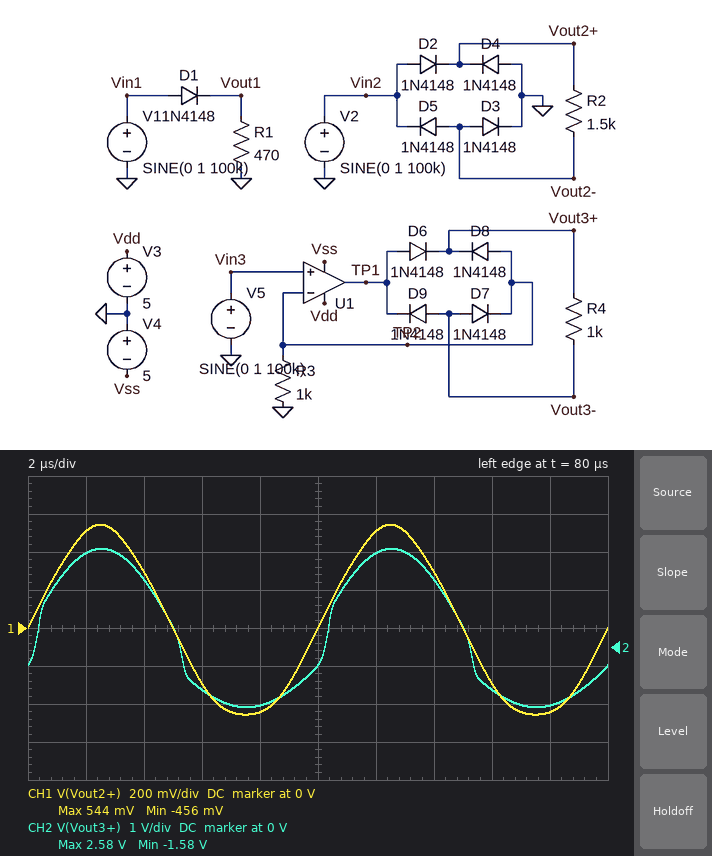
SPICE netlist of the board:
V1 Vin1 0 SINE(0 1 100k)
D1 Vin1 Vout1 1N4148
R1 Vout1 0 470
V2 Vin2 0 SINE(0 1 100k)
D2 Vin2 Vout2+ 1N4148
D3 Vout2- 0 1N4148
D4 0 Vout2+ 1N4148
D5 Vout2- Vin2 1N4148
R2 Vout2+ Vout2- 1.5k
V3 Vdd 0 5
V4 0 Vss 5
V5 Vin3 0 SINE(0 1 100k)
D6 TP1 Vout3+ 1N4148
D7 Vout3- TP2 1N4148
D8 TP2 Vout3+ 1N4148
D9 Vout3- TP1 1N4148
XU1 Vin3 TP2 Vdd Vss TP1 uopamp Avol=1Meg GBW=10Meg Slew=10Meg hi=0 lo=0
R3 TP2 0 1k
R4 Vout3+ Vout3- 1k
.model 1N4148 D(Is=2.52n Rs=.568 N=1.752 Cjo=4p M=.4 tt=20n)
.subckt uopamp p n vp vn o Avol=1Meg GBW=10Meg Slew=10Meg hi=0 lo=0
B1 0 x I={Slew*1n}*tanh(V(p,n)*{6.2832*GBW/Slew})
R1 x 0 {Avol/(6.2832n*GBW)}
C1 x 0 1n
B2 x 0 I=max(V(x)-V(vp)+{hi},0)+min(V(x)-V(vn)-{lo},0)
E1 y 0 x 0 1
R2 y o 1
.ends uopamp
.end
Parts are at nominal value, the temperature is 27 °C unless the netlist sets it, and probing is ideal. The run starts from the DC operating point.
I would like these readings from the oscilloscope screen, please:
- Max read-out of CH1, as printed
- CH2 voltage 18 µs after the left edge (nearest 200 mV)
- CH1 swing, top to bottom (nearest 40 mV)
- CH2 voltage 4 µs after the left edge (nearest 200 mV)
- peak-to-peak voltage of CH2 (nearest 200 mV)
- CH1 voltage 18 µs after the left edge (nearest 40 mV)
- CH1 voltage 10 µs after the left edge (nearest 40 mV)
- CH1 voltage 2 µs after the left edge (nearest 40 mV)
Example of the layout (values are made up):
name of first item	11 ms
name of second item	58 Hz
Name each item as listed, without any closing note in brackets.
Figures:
Max read-out of CH1, as printed	544 mV
CH2 voltage 18 µs after the left edge	-1.6 V
CH1 swing, top to bottom	1.00 V
CH2 voltage 4 µs after the left edge	1.8 V
peak-to-peak voltage of CH2	4.2 V
CH1 voltage 18 µs after the left edge	-440 mV
CH1 voltage 10 µs after the left edge	0 V
CH1 voltage 2 µs after the left edge	520 mV
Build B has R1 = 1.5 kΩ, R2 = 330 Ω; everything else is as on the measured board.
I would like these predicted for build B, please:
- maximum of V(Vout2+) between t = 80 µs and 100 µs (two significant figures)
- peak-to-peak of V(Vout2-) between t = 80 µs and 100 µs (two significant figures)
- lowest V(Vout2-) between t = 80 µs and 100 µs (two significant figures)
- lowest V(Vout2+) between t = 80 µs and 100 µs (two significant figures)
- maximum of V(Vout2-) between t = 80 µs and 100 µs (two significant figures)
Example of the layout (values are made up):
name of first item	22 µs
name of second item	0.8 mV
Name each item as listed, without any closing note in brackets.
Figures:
maximum of V(Vout2+) between t = 80 µs and 100 µs	520 mV
peak-to-peak of V(Vout2-) between t = 80 µs and 100 µs	1.0 V
lowest V(Vout2-) between t = 80 µs and 100 µs	-520 mV
lowest V(Vout2+) between t = 80 µs and 100 µs	-480 mV
maximum of V(Vout2-) between t = 80 µs and 100 µs	480 mV
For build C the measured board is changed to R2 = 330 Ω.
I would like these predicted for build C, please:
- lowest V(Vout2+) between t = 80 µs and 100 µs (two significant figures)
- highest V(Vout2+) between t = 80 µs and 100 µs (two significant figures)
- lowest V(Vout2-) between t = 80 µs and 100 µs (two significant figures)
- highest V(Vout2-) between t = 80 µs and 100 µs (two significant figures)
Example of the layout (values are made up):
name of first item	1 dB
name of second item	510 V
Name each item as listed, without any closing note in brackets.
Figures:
lowest V(Vout2+) between t = 80 µs and 100 µs	-480 mV
highest V(Vout2+) between t = 80 µs and 100 µs	520 mV
lowest V(Vout2-) between t = 80 µs and 100 µs	-520 mV
highest V(Vout2-) between t = 80 µs and 100 µs	480 mV
